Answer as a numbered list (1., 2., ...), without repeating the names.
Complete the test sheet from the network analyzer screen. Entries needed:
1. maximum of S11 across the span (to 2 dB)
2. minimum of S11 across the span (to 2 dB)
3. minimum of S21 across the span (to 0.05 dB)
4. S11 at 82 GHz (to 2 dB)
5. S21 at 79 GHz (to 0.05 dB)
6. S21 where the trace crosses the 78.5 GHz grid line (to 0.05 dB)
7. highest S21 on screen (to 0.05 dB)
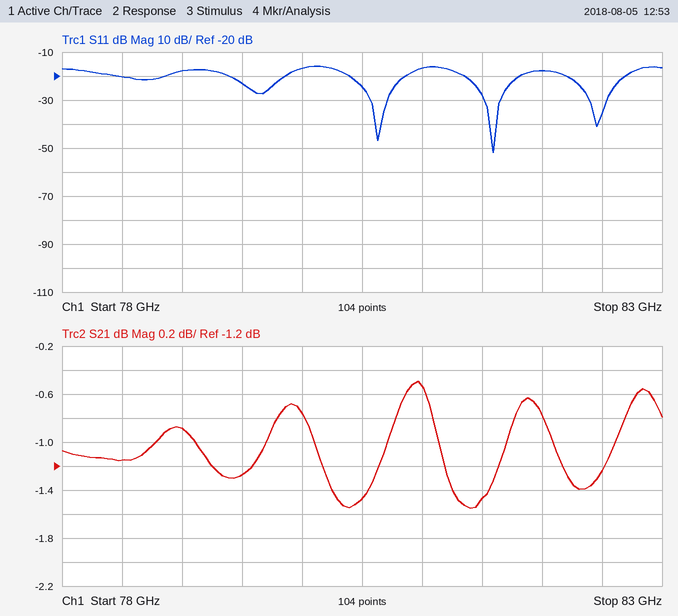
1. -16 dB
2. -52 dB
3. -1.55 dB
4. -18 dB
5. -0.90 dB
6. -1.15 dB
7. -0.50 dB
